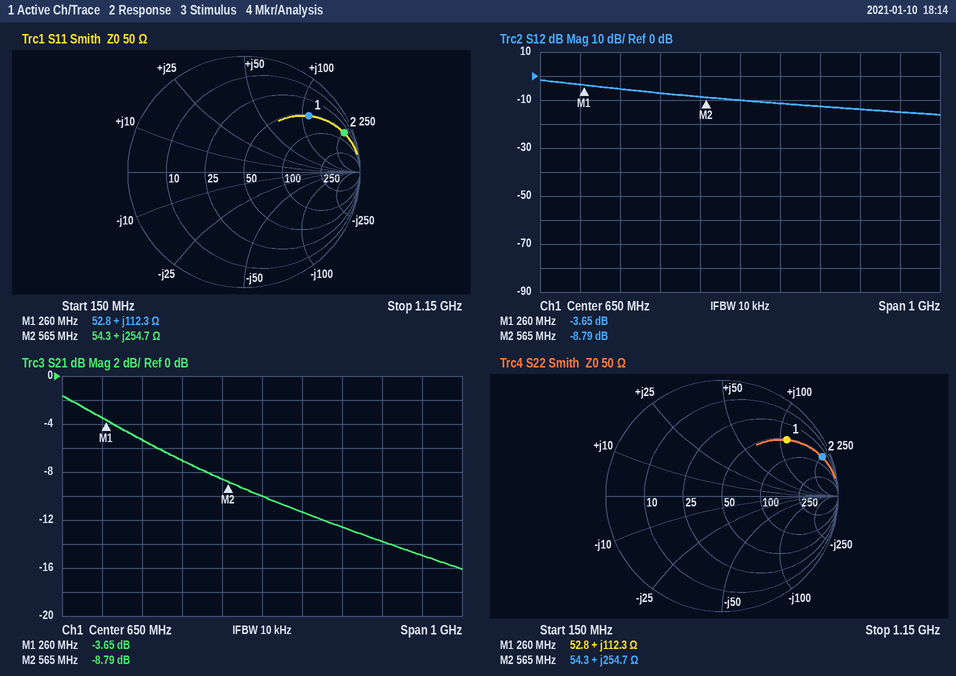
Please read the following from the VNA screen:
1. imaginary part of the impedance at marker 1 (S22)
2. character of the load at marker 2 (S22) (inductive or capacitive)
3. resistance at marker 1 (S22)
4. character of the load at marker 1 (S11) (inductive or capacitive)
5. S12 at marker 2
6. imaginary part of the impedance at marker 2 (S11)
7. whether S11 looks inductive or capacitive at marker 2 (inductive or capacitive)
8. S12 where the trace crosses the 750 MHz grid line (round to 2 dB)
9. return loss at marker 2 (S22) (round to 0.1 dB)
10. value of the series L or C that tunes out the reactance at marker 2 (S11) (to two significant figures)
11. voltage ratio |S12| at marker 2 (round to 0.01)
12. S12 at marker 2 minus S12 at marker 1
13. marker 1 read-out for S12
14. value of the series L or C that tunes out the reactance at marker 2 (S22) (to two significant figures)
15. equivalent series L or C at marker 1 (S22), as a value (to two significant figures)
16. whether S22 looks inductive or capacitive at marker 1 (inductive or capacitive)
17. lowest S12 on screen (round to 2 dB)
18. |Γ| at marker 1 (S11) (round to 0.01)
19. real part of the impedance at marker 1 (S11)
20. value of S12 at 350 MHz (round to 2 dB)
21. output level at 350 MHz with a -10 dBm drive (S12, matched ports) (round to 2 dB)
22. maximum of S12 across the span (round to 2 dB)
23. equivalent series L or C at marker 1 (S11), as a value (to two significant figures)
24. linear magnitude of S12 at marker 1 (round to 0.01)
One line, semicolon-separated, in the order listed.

+112.3 Ω; inductive; 52.8 Ω; inductive; -8.79 dB; +254.7 Ω; inductive; -12 dB; 0.7 dB; 1.1 pF; 0.36; -5.14 dB; -3.65 dB; 1.1 pF; 69 nH; inductive; -16 dB; 0.74; 52.8 Ω; -6 dB; -16 dBm; -2 dB; 69 nH; 0.66
